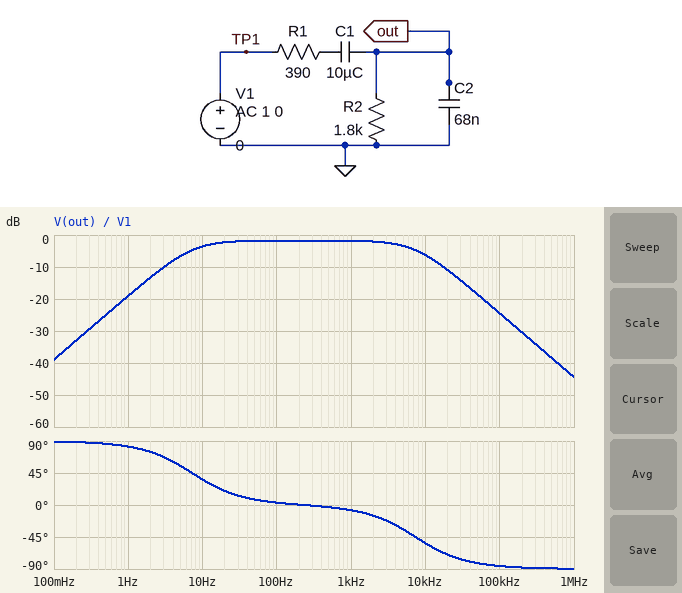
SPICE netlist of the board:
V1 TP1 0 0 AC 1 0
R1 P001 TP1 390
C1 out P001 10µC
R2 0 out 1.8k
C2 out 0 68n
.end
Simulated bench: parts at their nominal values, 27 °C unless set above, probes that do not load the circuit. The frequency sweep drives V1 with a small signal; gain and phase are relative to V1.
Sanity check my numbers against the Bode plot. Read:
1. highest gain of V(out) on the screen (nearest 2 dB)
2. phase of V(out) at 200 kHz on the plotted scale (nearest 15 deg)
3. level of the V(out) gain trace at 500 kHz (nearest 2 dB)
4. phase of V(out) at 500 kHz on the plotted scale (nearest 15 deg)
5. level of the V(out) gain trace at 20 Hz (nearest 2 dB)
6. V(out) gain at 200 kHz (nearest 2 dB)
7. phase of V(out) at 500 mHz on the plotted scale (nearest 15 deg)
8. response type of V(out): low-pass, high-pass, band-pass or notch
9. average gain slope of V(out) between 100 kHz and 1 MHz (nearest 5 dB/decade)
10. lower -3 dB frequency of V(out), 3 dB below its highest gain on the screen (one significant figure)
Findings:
-2 dB
-90 deg
-38 dB
-90 deg
-2 dB
-30 dB
90 deg
band-pass
-20 dB/decade
7 Hz
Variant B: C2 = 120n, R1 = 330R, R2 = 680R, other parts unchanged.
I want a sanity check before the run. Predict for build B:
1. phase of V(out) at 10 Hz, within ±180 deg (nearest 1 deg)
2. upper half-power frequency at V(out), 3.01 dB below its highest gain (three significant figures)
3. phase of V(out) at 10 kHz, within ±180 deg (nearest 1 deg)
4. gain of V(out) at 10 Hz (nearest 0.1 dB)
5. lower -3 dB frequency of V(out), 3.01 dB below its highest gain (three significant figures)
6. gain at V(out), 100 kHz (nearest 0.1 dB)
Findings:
57 deg
6.03 kHz
-59 deg
-8.9 dB
15.6 Hz
-27.9 dB
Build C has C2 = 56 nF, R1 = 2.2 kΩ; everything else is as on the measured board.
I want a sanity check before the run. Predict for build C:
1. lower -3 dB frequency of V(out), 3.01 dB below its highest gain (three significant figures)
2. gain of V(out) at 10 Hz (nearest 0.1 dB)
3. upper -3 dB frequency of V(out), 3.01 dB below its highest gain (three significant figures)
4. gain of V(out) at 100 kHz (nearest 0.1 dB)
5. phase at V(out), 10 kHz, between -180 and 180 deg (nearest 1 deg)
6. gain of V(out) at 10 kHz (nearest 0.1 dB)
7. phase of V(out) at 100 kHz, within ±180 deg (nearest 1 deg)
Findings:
3.96 Hz
-7.6 dB
2.88 kHz
-37.8 dB
-74 deg
-18.1 dB
-88 deg
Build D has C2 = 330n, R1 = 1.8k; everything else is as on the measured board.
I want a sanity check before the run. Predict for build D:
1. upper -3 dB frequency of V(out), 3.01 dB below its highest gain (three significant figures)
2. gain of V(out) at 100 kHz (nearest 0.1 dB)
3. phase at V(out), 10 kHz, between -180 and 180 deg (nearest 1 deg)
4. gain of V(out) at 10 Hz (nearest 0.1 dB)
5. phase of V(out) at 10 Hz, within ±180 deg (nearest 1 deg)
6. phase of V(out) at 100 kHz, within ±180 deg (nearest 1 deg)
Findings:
549 Hz
-51.4 dB
-87 deg
-6.9 dB
23 deg
-90 deg
